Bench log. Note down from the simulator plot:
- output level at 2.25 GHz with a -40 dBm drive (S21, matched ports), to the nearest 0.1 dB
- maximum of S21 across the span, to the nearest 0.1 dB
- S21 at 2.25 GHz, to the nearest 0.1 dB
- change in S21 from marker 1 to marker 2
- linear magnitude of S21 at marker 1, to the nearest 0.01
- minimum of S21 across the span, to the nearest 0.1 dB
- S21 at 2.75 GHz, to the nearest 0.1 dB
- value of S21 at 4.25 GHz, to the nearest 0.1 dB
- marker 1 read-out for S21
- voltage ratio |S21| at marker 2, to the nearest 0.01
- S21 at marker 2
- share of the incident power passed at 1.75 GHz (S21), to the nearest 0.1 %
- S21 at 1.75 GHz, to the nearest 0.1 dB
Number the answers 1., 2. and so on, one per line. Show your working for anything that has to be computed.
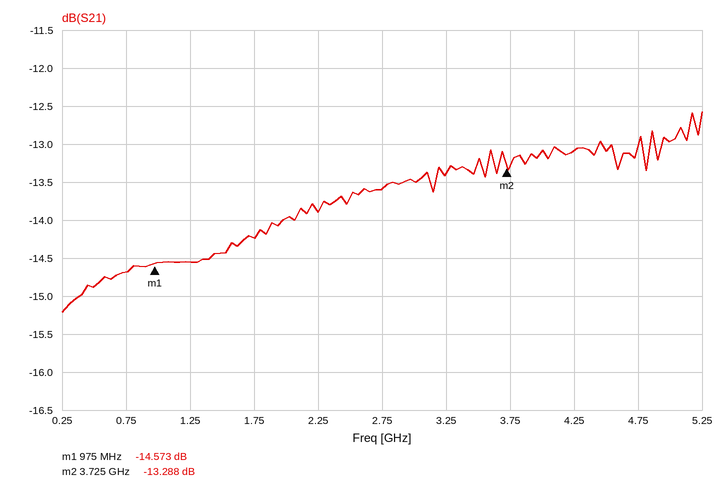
1. -40 dBm + (-13.9 dB) = -53.9 dBm
2. -12.6 dB
3. -13.9 dB
4. -13.288 − (-14.573) = 1.285 dB
5. 10^(-14.573/20) ≈ 0.19
6. -15.2 dB
7. -13.6 dB
8. -13.1 dB
9. -14.573 dB
10. 10^(-13.288/20) ≈ 0.22
11. -13.288 dB
12. 10^(-14.2/10) ≈ 3.8 %
13. -14.2 dB
